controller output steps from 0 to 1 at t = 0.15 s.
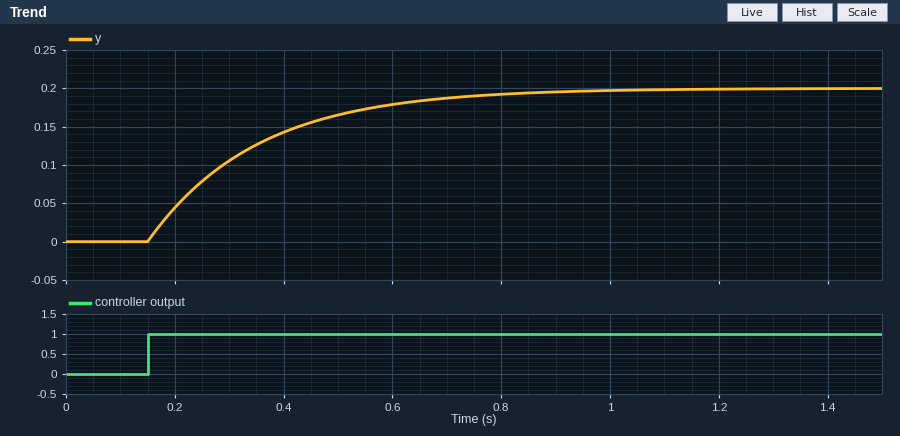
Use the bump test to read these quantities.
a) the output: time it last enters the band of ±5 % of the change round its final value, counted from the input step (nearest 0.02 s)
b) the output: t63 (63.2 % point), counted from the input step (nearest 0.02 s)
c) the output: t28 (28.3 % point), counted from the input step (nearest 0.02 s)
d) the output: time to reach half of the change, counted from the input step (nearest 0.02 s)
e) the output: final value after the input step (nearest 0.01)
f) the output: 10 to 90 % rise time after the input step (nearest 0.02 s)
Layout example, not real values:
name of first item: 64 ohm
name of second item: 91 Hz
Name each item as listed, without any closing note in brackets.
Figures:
the output: time it last enters the band of ±5 % of the change round its final value, counted from the input step: 0.60 s
the output: t63 (63.2 % point), counted from the input step: 0.20 s
the output: t28 (28.3 % point), counted from the input step: 0.06 s
the output: time to reach half of the change, counted from the input step: 0.14 s
the output: final value after the input step: 0.20
the output: 10 to 90 % rise time after the input step: 0.44 s
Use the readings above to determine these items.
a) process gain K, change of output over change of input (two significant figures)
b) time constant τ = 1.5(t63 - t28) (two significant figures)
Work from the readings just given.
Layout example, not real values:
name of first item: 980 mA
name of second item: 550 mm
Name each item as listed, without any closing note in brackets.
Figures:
process gain K, change of output over change of input: 0.20
time constant τ = 1.5(t63 - t28): 0.21 s
